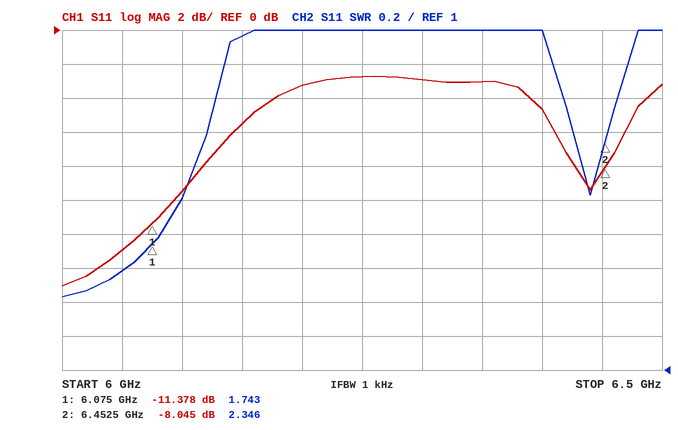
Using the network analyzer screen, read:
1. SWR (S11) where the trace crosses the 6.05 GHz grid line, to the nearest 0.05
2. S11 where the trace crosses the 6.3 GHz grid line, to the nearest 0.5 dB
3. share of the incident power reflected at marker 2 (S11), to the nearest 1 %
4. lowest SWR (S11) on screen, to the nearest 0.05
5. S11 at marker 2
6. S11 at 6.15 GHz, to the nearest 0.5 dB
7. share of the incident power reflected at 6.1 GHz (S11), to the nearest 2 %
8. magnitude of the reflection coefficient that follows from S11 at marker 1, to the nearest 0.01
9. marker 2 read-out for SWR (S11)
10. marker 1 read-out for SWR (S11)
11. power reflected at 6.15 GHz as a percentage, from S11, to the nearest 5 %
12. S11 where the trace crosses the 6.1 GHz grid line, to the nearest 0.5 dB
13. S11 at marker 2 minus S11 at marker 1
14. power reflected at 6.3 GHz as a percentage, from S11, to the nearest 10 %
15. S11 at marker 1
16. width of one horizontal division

1.60
-3.0 dB
16 %
1.45
-8.045 dB
-5.5 dB
12 %
0.27
2.346
1.743
30 %
-9.5 dB
3.333 dB
50 %
-11.378 dB
50 MHz
